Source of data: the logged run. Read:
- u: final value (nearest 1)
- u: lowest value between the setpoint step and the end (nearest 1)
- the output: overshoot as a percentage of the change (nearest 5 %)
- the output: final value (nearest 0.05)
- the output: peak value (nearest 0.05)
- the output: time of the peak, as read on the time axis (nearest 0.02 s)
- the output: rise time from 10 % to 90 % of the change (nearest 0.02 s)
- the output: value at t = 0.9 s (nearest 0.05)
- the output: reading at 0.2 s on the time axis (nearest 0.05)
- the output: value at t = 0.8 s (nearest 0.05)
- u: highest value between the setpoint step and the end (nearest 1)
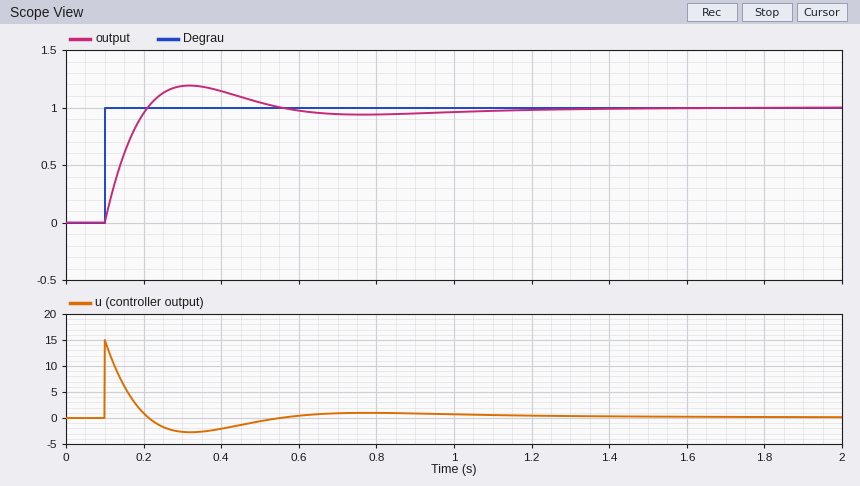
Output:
0
-3
20 %
1.00
1.20
0.32 s
0.08 s
0.95
0.95
0.95
15
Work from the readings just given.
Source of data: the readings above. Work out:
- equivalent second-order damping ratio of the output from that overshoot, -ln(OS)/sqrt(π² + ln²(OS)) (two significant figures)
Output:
0.46
